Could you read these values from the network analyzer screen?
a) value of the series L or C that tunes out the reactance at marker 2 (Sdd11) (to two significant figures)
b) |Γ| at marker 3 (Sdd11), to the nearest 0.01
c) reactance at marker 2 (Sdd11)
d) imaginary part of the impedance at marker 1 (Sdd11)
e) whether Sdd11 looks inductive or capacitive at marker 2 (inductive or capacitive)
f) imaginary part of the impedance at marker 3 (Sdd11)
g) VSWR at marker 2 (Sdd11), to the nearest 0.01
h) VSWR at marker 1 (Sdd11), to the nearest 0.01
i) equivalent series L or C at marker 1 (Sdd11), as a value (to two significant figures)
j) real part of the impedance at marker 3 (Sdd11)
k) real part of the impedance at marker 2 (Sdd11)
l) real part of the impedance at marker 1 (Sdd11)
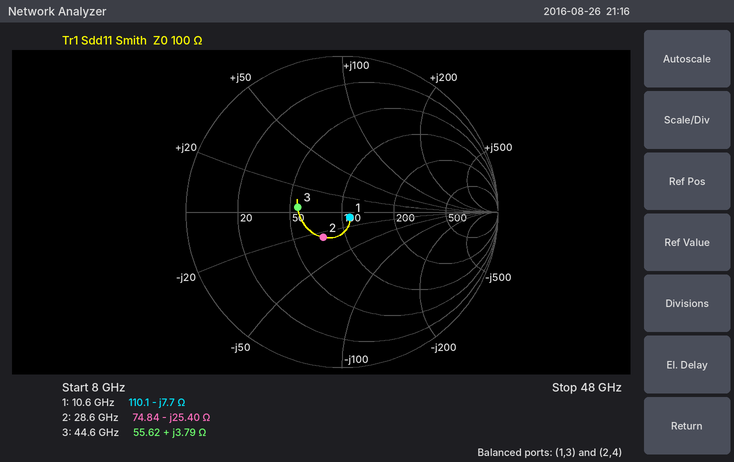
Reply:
140 pH
0.29
-25.40 Ω
-7.7 Ω
capacitive
+3.79 Ω
1.51
1.13
1.9 pF
55.62 Ω
74.84 Ω
110.1 Ω
